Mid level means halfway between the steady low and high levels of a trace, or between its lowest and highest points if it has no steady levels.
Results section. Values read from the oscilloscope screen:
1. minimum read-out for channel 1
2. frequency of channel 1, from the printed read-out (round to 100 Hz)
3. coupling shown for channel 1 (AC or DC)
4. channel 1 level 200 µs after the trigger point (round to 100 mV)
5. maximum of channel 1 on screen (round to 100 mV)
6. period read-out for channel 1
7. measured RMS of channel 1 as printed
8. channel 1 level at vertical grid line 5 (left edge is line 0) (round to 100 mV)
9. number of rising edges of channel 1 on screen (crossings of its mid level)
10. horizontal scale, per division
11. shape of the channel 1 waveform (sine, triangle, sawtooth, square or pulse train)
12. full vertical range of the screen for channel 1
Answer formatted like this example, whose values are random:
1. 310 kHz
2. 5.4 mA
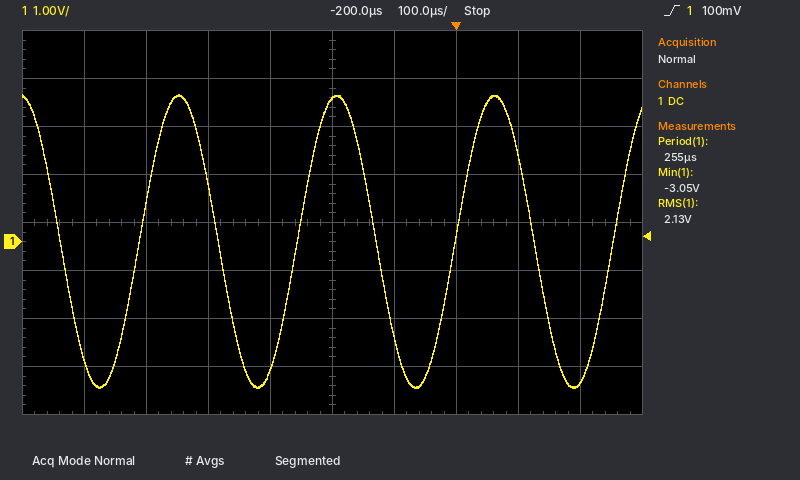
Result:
1. -3.05 V
2. 3.9 kHz
3. DC
4. -2.9 V
5. 3.1 V
6. 255 µs
7. 2.13 V
8. 3.0 V
9. 4
10. 100 µs
11. sine
12. 8 V
